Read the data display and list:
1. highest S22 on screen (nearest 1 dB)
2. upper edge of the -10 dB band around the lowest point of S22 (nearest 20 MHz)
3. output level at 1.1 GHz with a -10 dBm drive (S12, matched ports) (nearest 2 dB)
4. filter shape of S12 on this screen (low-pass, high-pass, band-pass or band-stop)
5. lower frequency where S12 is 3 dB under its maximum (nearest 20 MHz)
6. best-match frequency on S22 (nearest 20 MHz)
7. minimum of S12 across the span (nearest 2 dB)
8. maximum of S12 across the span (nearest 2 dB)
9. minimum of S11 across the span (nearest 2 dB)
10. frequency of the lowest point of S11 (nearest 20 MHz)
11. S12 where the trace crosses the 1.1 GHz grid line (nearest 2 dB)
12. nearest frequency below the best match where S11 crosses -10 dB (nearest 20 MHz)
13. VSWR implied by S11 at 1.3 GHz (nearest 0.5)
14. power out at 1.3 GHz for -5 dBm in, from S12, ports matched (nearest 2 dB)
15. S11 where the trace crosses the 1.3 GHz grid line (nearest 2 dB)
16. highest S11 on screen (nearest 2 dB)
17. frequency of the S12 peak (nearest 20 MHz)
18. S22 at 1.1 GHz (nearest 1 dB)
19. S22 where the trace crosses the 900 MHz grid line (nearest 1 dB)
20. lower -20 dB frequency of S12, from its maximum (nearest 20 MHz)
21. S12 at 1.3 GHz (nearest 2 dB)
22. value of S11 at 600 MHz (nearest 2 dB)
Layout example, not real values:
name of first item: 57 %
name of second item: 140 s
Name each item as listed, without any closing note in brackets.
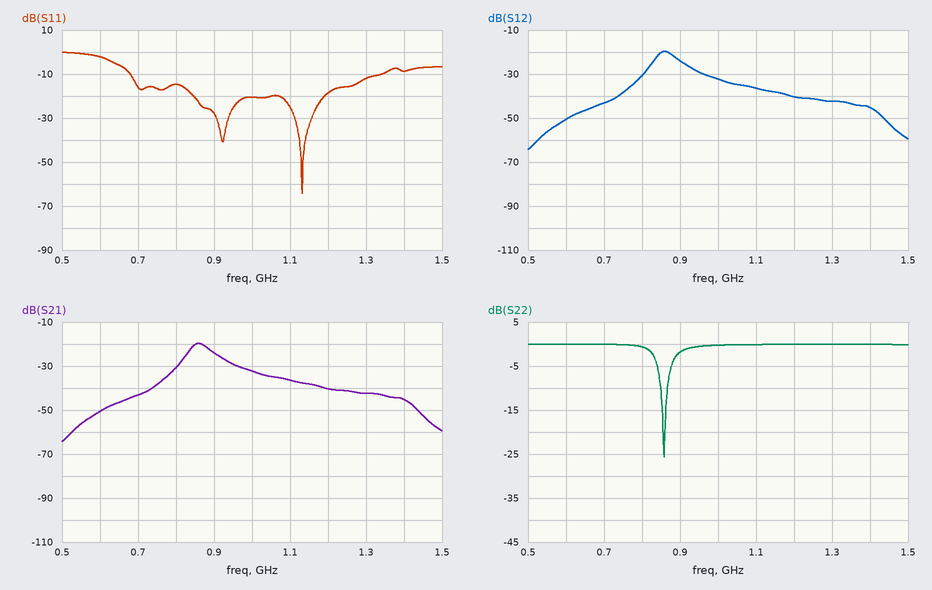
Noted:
highest S22 on screen: 0 dB
upper edge of the -10 dB band around the lowest point of S22: 860 MHz
output level at 1.1 GHz with a -10 dBm drive (S12, matched ports): -46 dBm
filter shape of S12 on this screen: band-pass
lower frequency where S12 is 3 dB under its maximum: 840 MHz
best-match frequency on S22: 860 MHz
minimum of S12 across the span: -64 dB
maximum of S12 across the span: -20 dB
minimum of S11 across the span: -64 dB
frequency of the lowest point of S11: 1.14 GHz
S12 where the trace crosses the 1.1 GHz grid line: -36 dB
nearest frequency below the best match where S11 crosses -10 dB: 680 MHz
VSWR implied by S11 at 1.3 GHz: 1.5
power out at 1.3 GHz for -5 dBm in, from S12, ports matched: -48 dBm
S11 where the trace crosses the 1.3 GHz grid line: -12 dB
highest S11 on screen: 0 dB
frequency of the S12 peak: 860 MHz
S22 at 1.1 GHz: 0 dB
S22 where the trace crosses the 900 MHz grid line: -2 dB
lower -20 dB frequency of S12, from its maximum: 740 MHz
S12 at 1.3 GHz: -42 dB
value of S11 at 600 MHz: -2 dB
